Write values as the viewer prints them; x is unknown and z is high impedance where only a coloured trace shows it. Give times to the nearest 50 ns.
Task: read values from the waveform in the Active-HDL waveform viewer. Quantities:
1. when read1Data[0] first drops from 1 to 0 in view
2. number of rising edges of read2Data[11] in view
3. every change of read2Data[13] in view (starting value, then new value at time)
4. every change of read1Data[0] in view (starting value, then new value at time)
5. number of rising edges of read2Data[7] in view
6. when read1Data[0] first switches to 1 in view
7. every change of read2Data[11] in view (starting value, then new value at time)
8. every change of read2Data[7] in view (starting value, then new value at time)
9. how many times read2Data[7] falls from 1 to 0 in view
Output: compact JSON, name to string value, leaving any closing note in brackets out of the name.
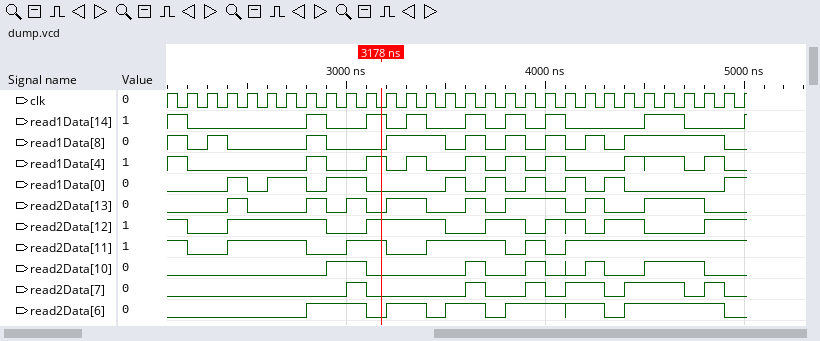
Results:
{"when read1Data[0] first drops from 1 to 0 in view": "2500 ns", "number of rising edges of read2Data[11] in view": "5", "every change of read2Data[13] in view": "0, 1 at 2400 ns, 0 at 2500 ns, 1 at 2800 ns, 0 at 2900 ns, 1 at 3000 ns, 0 at 3100 ns, 1 at 3200 ns, 0 at 3400 ns, 1 at 3600 ns, 0 at 3700 ns, 1 at 3800 ns, 0 at 4100 ns, 1 at 4200 ns, 0 at 4300 ns, 1 at 4500 ns, 0 at 4800 ns", "every change of read1Data[0] in view": "0, 1 at 2400 ns, 0 at 2500 ns, 1 at 2600 ns, 0 at 2800 ns, 1 at 2900 ns, 0 at 3100 ns, 1 at 3500 ns, 0 at 3600 ns, 1 at 3700 ns, 0 at 3800 ns, 1 at 3900 ns, 0 at 4000 ns, 1 at 4100 ns, 0 at 4200 ns, 1 at 4300 ns, 0 at 4400 ns, 1 at 4900 ns", "number of rising edges of read2Data[7] in view": "6", "when read1Data[0] first switches to 1 in view": "2400 ns", "every change of read2Data[11] in view": "1, 0 at 2200 ns, 1 at 2400 ns, 0 at 2800 ns, 1 at 3000 ns, 0 at 3200 ns, 1 at 3400 ns, 0 at 3800 ns, 1 at 3900 ns, 0 at 4000 ns, 1 at 4100 ns", "every change of read2Data[7] in view": "0, 1 at 3000 ns, 0 at 3100 ns, 1 at 3600 ns, 0 at 3700 ns, 1 at 3900 ns, 0 at 4000 ns, 1 at 4100 ns, 0 at 4300 ns, 1 at 4400 ns, 0 at 4700 ns, 1 at 4800 ns, 0 at 4900 ns", "how many times read2Data[7] falls from 1 to 0 in view": "6"}
